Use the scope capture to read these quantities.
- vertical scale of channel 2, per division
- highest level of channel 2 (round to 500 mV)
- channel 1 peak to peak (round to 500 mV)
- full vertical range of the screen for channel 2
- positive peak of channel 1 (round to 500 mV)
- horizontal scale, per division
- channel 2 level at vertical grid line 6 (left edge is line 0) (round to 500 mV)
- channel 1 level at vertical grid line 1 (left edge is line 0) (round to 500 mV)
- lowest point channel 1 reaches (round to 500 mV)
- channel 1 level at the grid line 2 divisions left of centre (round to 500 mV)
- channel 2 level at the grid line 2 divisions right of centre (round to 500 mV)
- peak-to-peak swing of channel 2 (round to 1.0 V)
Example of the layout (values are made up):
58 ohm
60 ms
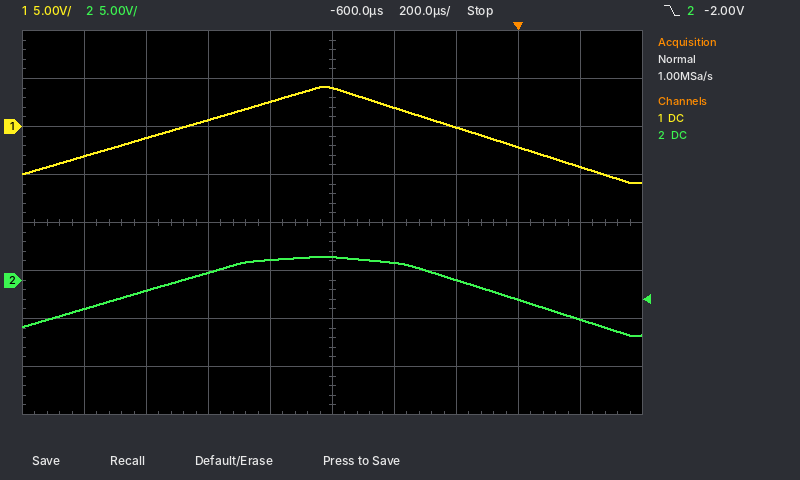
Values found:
5 V
2.5 V
10.0 V
40 V
4.0 V
200 µs
2.0 V
-3.0 V
-6.0 V
500 mV
0.0 V
8.0 V
